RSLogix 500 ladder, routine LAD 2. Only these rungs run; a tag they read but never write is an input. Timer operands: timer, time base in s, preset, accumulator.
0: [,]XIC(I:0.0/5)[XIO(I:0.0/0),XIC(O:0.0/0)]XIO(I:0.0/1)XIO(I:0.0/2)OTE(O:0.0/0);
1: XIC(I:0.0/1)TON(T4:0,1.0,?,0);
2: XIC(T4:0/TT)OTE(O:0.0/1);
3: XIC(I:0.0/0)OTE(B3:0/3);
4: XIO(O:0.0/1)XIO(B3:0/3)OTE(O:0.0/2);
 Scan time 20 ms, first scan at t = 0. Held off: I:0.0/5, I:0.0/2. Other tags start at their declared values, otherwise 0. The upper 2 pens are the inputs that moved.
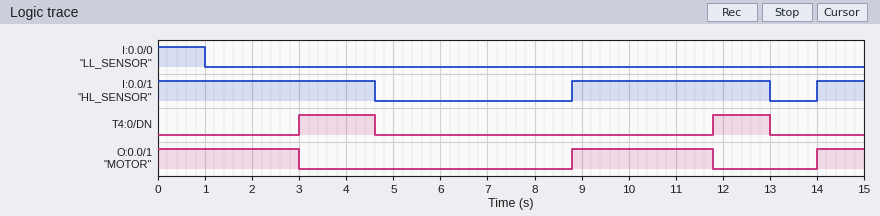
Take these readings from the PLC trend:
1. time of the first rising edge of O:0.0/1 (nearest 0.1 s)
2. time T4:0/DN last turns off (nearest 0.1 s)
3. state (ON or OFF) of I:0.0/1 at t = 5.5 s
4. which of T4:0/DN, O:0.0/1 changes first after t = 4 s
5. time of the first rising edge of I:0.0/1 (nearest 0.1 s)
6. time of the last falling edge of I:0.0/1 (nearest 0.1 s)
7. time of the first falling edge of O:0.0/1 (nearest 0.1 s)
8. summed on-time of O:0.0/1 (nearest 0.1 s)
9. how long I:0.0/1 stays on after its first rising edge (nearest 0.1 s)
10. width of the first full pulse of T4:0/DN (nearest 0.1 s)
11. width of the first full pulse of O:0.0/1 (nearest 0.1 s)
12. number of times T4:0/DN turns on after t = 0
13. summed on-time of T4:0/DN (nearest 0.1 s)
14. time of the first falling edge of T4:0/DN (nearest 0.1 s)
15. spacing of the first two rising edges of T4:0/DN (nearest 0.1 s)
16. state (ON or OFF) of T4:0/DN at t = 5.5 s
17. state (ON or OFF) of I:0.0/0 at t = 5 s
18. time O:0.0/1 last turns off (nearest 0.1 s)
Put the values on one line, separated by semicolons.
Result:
8.8 s; 13.0 s; OFF; T4:0/DN; 8.8 s; 13.0 s; 3.0 s; 7.0 s; 4.2 s; 1.6 s; 3.0 s; 2; 2.8 s; 4.6 s; 8.8 s; OFF; OFF; 11.8 s
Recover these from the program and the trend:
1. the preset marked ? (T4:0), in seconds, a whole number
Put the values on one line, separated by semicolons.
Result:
3 s
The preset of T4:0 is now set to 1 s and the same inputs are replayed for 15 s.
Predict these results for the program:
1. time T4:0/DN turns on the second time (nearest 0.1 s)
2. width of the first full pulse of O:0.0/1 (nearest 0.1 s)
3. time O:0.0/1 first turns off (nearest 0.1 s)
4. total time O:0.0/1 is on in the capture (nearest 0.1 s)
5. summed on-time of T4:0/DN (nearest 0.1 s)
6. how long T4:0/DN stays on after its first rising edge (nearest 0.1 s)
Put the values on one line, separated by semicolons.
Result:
9.8 s; 1.0 s; 1.0 s; 3.0 s; 6.8 s; 3.6 s
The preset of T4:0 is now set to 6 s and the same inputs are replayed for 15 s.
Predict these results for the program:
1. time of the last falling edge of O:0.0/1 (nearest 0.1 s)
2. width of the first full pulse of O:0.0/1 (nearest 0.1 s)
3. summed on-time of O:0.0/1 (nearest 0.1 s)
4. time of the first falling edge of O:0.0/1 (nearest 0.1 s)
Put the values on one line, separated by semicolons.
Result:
13.0 s; 4.2 s; 9.8 s; 4.6 s
